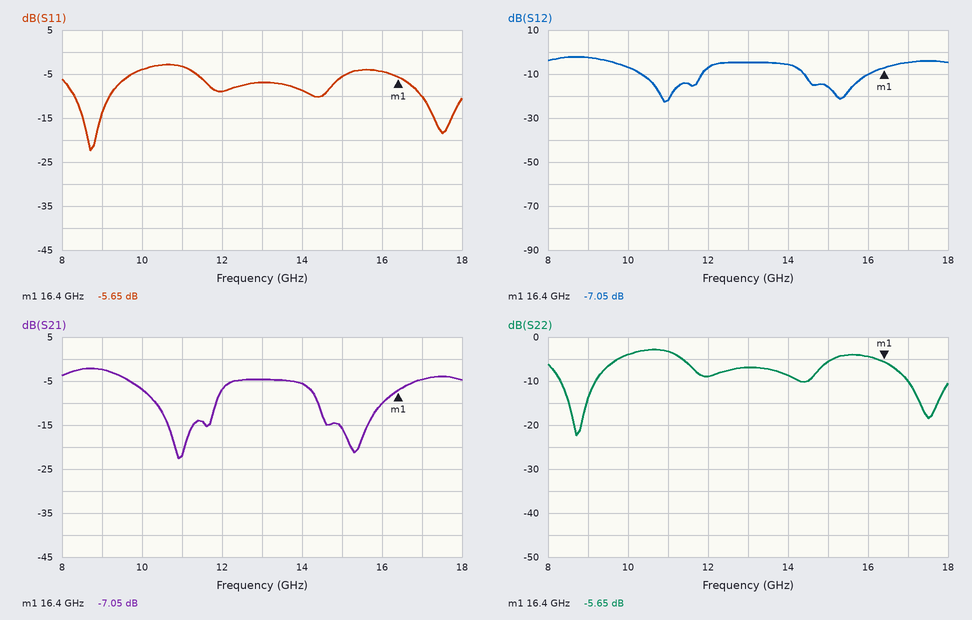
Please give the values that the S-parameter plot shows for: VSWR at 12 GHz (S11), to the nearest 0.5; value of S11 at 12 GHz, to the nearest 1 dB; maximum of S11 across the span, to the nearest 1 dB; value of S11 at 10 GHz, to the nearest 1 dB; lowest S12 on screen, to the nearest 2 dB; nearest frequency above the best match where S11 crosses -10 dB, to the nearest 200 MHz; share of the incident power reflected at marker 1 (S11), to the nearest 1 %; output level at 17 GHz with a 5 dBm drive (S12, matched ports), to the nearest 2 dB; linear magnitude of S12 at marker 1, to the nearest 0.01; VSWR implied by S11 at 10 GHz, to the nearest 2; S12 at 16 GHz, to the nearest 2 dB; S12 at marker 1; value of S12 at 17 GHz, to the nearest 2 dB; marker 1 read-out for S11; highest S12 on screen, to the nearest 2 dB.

2.0
-9 dB
-3 dB
-4 dB
-22 dB
9.2 GHz
27 %
0 dBm
0.44
4
-10 dB
-7.05 dB
-4 dB
-5.65 dB
-2 dB
